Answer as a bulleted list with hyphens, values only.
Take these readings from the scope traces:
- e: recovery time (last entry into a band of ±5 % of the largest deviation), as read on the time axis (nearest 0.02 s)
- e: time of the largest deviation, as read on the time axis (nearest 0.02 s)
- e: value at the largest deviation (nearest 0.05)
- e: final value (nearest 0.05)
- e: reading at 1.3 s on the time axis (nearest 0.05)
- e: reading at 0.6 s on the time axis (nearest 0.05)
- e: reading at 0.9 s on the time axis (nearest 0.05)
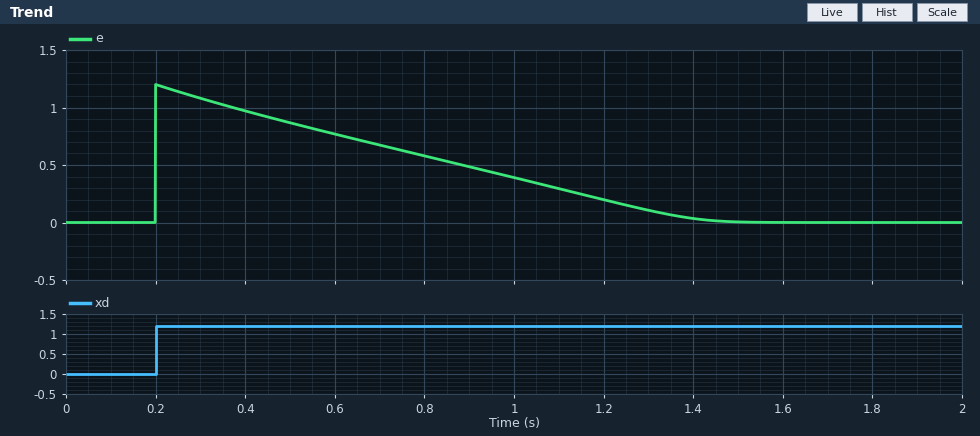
- 1.36 s
- 0.20 s
- 1.20
- 0.00
- 0.10
- 0.75
- 0.50
